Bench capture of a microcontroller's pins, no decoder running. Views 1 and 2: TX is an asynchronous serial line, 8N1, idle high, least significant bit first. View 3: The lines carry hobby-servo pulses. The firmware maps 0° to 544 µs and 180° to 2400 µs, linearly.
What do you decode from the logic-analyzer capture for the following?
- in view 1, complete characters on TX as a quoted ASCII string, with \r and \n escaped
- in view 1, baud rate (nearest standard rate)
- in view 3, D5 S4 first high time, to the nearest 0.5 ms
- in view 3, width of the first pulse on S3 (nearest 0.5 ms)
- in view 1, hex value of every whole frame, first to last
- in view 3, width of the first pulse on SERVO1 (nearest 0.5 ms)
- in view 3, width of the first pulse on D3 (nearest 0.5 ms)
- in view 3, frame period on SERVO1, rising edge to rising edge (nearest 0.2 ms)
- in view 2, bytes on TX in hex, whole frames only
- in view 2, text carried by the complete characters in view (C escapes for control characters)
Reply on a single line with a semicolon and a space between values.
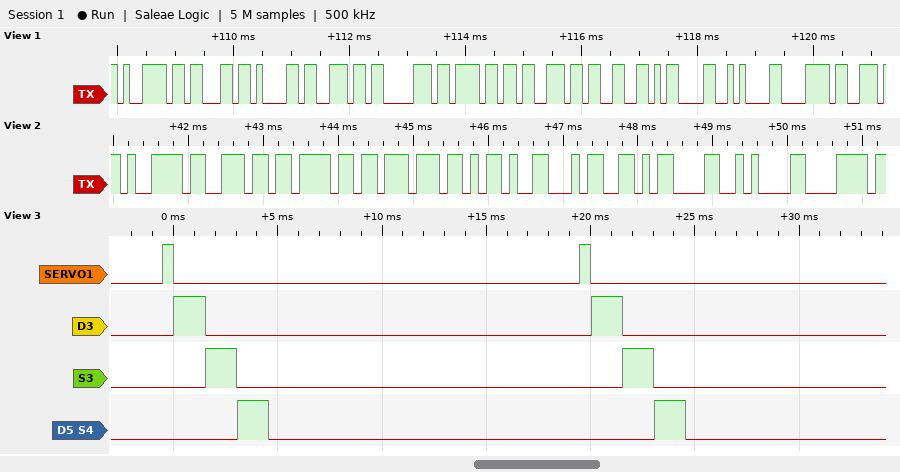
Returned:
"ycanpos3\r\nx"; 9600 baud; 1.5 ms; 1.5 ms; 79 63 61 6E 70 6F 73 33 0D 0A 78; 0.5 ms; 1.5 ms; 20.0 ms; 79 6E 6F 77 2D 34 0D 0A 78; "ynow-4\r\nx"
